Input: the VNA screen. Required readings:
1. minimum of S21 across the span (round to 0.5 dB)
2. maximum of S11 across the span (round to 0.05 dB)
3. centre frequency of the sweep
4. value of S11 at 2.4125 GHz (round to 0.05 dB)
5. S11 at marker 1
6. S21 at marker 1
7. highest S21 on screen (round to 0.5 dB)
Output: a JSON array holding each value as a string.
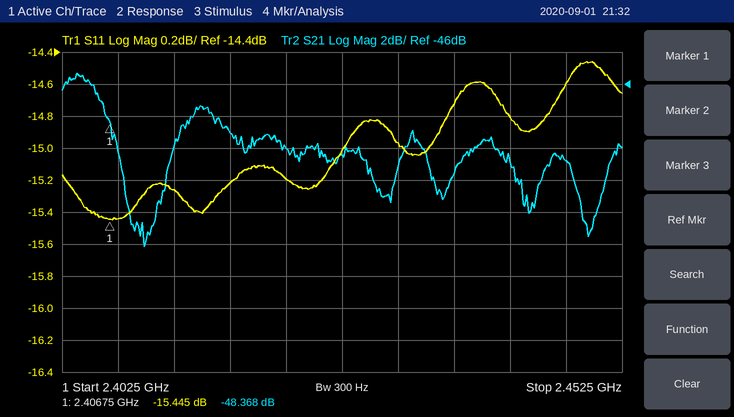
["-56.0 dB", "-14.45 dB", "2.4275 GHz", "-15.25 dB", "-15.445 dB", "-48.368 dB", "-45.5 dB"]
